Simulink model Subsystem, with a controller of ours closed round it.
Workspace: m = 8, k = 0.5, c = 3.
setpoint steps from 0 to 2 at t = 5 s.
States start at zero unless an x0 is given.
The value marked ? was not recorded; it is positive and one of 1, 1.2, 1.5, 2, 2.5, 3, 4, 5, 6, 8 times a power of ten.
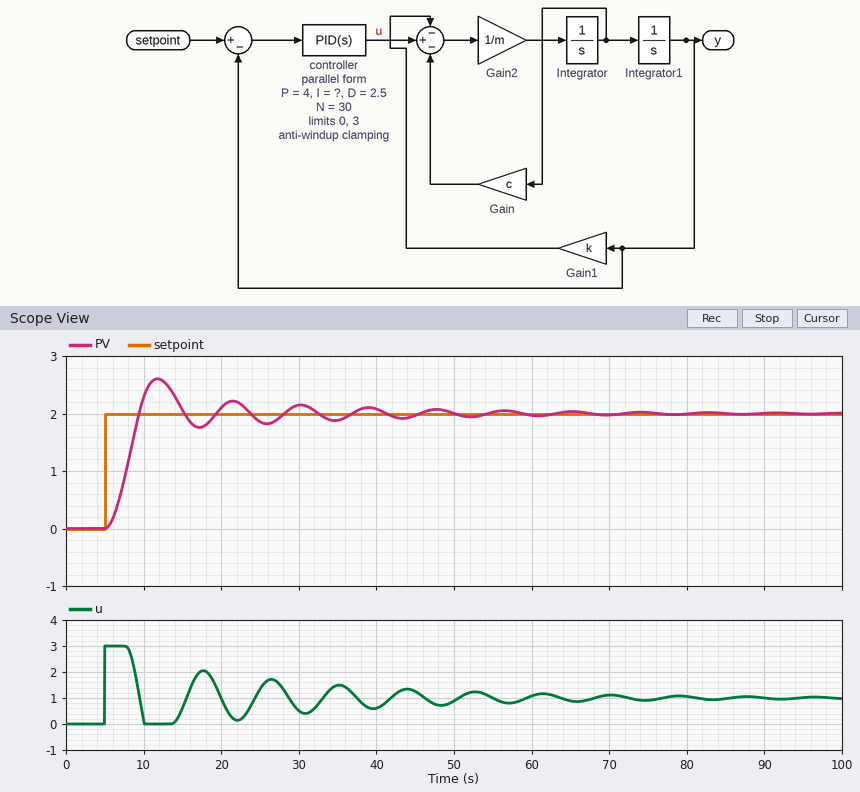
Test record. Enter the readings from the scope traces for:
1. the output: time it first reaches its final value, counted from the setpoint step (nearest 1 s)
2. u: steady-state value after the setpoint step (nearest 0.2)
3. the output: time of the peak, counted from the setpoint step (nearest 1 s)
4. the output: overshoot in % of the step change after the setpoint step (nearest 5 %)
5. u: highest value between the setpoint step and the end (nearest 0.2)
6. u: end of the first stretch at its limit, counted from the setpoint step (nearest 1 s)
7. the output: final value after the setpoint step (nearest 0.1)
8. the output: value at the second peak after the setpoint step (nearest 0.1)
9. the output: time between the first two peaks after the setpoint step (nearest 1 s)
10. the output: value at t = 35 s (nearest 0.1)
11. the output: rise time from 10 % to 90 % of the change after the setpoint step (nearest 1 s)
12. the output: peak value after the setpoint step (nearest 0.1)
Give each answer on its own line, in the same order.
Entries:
4 s
1.0
7 s
30 %
3.0
3 s
2.0
2.2
10 s
1.9
3 s
2.6
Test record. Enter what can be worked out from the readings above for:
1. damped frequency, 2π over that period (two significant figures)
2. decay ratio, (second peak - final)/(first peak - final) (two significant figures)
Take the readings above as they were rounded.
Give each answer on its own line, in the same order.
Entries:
0.63 rad/s
0.33
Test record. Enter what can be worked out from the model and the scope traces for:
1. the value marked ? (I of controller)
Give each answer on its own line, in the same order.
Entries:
2.5
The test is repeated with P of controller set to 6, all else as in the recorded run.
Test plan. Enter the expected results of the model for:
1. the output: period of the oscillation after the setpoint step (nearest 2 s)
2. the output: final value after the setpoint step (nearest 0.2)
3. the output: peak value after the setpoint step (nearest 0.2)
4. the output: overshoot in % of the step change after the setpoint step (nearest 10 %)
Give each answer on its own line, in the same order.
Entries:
8 s
2.0
2.4
20 %
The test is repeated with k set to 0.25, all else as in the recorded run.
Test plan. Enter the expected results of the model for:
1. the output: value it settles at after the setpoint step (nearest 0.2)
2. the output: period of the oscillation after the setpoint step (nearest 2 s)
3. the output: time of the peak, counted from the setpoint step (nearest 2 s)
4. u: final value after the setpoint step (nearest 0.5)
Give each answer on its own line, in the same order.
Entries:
2.0
12 s
8 s
0.5
